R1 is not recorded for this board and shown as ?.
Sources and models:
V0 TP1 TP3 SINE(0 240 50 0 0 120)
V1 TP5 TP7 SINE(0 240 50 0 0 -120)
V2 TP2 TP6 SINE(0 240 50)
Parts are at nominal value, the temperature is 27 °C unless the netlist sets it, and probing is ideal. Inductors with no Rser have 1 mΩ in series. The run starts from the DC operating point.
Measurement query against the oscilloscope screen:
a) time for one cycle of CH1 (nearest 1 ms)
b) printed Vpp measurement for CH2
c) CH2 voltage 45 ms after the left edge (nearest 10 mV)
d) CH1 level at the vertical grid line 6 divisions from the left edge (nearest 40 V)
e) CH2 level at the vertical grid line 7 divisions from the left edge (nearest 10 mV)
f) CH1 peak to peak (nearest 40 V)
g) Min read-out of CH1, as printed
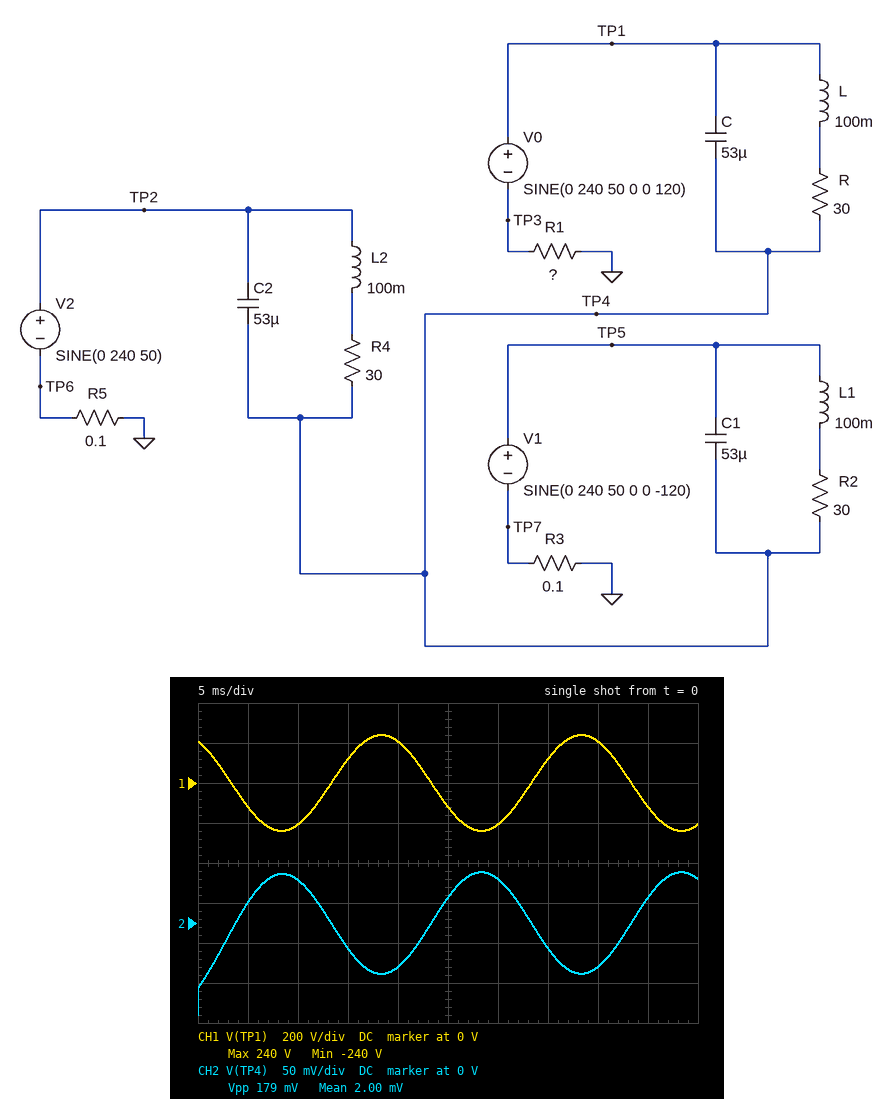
20 ms
179 mV
30 mV
-200 V
-30 mV
480 V
-240 V
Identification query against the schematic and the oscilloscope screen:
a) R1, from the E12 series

0.15 Ω
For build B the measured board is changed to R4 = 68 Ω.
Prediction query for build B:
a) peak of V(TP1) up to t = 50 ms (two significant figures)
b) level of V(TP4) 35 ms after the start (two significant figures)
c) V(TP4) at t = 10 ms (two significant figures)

240 V
4.9 V
-51 V
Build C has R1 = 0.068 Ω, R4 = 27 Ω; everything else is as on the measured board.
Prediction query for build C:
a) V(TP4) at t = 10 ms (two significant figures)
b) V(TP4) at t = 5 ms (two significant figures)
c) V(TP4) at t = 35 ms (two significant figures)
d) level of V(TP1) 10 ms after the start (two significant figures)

7.1 V
1.7 V
580 mV
-210 V
